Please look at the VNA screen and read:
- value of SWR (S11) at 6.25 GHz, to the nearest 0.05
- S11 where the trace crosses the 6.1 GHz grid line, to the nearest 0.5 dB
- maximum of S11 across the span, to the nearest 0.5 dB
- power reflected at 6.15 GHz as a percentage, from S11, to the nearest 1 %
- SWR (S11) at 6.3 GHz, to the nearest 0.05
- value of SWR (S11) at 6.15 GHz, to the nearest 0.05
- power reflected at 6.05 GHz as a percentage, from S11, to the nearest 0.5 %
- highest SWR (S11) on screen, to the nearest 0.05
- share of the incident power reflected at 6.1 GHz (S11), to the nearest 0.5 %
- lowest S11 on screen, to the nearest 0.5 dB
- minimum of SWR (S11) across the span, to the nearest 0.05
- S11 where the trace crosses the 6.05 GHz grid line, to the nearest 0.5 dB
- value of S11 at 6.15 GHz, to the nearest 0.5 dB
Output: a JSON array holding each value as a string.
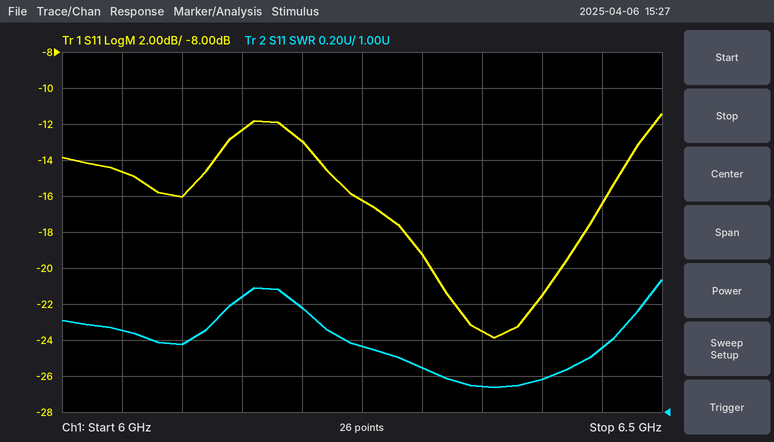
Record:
["1.35", "-16.0 dB", "-11.5 dB", "6 %", "1.25", "1.65", "3.5 %", "1.75", "2.5 %", "-24.0 dB", "1.15", "-14.5 dB", "-12.5 dB"]
